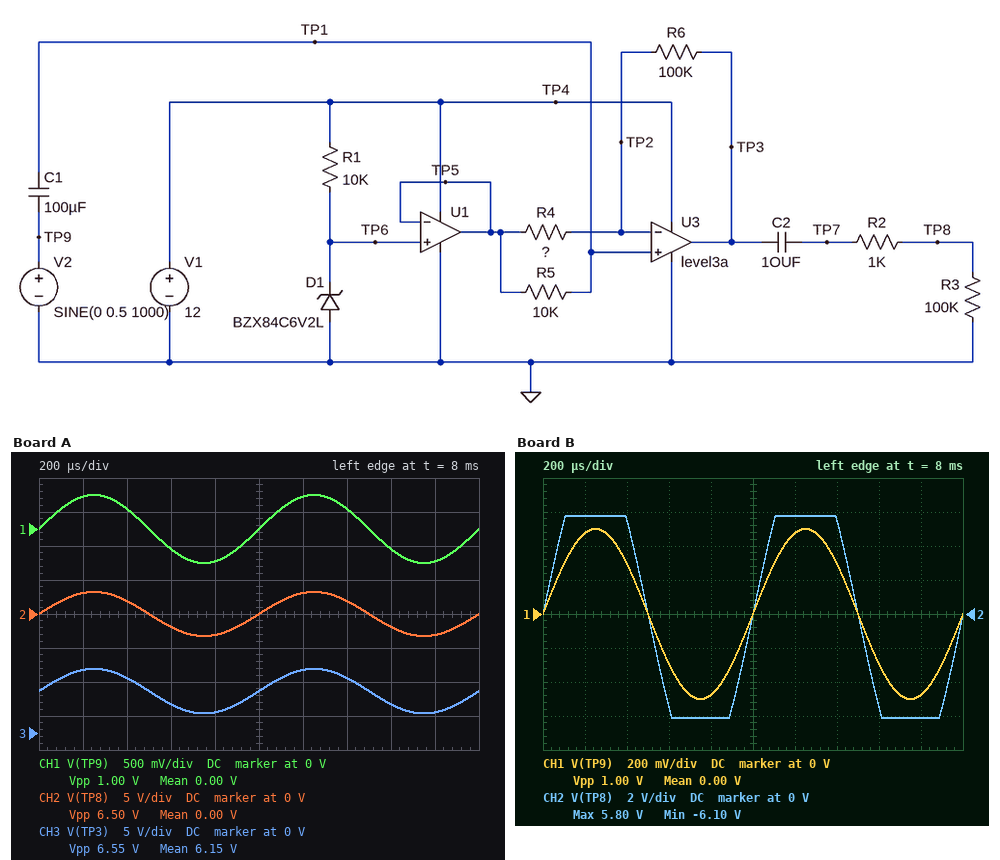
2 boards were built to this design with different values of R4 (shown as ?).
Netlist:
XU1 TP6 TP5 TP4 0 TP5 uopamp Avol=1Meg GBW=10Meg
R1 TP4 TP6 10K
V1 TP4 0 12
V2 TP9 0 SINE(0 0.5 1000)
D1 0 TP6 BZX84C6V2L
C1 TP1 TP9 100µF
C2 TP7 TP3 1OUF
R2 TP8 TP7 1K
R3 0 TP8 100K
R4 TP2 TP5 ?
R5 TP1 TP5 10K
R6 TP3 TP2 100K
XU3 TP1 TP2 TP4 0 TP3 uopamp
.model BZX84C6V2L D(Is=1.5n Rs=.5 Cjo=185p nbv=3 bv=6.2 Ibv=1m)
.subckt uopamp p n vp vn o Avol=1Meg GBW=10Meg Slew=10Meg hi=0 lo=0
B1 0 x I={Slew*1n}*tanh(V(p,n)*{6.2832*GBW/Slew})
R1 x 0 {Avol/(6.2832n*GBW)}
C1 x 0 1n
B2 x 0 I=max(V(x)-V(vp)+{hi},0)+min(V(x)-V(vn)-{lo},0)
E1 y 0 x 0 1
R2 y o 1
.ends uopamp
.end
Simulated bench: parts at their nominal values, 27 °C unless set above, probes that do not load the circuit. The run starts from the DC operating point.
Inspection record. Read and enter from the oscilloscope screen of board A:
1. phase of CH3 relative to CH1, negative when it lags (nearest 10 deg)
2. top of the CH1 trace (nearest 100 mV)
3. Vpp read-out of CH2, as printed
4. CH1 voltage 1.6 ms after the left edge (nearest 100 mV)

0 deg
500 mV
6.50 V
-300 mV
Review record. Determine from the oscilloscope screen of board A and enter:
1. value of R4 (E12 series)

18 kΩ
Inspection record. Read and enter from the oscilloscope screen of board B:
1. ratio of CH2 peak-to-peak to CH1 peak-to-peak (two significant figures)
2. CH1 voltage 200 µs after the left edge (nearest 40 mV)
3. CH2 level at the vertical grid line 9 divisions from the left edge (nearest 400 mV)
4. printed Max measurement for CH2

12
480 mV
-6.0 V
5.80 V
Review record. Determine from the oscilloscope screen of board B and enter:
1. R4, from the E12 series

5.6 kΩ
